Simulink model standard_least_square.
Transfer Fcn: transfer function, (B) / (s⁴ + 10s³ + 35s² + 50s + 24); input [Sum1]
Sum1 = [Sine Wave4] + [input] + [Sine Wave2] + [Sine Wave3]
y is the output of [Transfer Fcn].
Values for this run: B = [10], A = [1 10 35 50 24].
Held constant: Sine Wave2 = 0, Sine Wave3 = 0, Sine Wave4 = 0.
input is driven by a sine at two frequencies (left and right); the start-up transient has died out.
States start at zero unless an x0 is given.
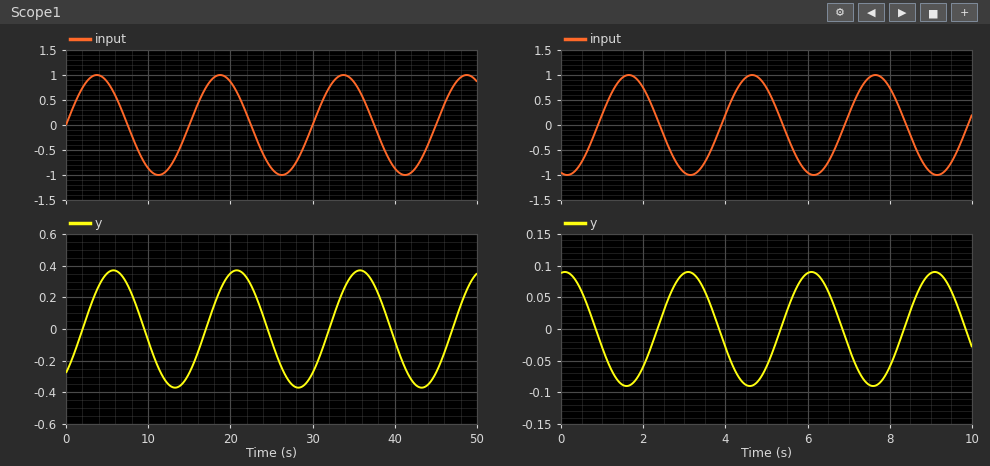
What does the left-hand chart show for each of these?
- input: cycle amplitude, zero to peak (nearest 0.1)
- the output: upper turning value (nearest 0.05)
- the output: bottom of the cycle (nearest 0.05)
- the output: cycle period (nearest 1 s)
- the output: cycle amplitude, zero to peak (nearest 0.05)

1.0
0.35
-0.35
15 s
0.35
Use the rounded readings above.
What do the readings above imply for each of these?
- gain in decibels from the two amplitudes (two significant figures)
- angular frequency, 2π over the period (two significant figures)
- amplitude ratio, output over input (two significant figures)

-9.1 dB
0.42 rad/s
0.35
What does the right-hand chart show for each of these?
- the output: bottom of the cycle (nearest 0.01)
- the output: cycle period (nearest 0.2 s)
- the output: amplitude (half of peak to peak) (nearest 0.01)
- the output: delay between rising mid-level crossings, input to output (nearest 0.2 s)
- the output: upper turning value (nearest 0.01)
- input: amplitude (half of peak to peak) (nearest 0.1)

-0.09
3.0 s
0.09
1.4 s
0.09
1.0
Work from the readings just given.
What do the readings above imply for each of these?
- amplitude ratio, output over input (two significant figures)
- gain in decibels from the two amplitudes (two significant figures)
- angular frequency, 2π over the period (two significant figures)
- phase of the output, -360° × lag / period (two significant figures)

0.090
-21 dB
2.1 rad/s
-170°
